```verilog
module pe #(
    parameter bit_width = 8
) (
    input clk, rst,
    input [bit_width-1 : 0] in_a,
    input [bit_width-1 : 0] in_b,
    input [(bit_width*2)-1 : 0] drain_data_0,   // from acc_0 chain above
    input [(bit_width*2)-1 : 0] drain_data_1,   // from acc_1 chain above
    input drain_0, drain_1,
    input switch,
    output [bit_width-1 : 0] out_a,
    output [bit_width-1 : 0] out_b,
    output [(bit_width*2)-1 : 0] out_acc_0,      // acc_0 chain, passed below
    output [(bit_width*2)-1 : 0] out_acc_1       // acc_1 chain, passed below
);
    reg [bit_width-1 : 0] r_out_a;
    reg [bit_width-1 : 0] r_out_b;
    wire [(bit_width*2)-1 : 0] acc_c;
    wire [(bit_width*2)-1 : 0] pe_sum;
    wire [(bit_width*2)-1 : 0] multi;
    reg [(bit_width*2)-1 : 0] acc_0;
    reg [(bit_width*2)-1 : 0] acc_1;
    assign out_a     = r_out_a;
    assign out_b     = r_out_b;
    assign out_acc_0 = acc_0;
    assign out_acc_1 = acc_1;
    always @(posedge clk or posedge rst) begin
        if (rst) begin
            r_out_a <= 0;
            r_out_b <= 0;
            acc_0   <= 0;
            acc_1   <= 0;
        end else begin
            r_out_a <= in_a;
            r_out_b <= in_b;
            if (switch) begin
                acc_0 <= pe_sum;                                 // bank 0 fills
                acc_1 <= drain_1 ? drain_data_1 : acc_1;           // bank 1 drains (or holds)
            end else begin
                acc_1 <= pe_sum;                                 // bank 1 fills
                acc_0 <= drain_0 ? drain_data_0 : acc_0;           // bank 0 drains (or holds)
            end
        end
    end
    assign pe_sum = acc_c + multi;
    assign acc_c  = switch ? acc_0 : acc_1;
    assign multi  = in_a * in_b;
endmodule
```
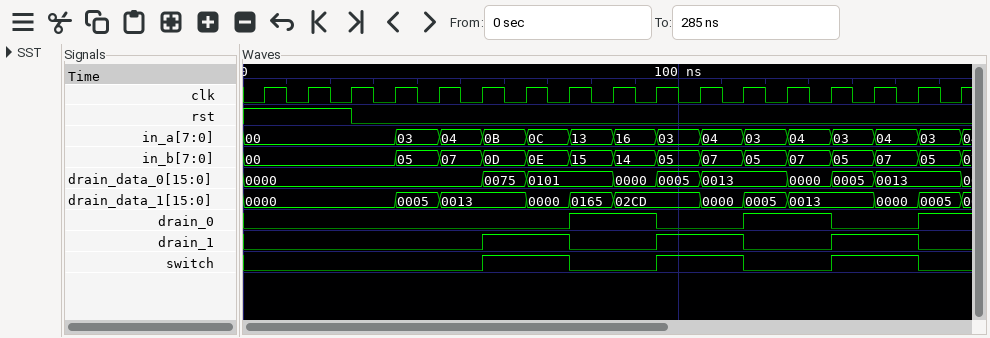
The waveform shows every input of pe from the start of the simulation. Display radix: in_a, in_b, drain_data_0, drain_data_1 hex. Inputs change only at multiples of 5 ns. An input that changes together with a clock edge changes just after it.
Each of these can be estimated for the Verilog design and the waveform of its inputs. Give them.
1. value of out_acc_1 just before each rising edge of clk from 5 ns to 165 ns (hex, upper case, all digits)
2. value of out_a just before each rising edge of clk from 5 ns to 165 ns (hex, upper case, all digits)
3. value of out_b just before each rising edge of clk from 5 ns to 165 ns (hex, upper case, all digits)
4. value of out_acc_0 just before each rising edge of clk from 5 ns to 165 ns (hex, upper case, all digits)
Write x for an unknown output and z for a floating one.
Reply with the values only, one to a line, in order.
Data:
0000, 0000, 0000, 0000, 0000, 000F, 002B, 0013, 0000, 018F, 0347, 02CD, 0000, 000F, 002B, 0013, 0000
00, 00, 00, 00, 00, 03, 04, 0B, 0C, 13, 16, 03, 04, 03, 04, 03, 04
00, 00, 00, 00, 00, 05, 07, 0D, 0E, 15, 14, 05, 07, 05, 07, 05, 07
0000, 0000, 0000, 0000, 0000, 0000, 0000, 008F, 0137, 0101, 0000, 000F, 002B, 0013, 0000, 000F, 002B
